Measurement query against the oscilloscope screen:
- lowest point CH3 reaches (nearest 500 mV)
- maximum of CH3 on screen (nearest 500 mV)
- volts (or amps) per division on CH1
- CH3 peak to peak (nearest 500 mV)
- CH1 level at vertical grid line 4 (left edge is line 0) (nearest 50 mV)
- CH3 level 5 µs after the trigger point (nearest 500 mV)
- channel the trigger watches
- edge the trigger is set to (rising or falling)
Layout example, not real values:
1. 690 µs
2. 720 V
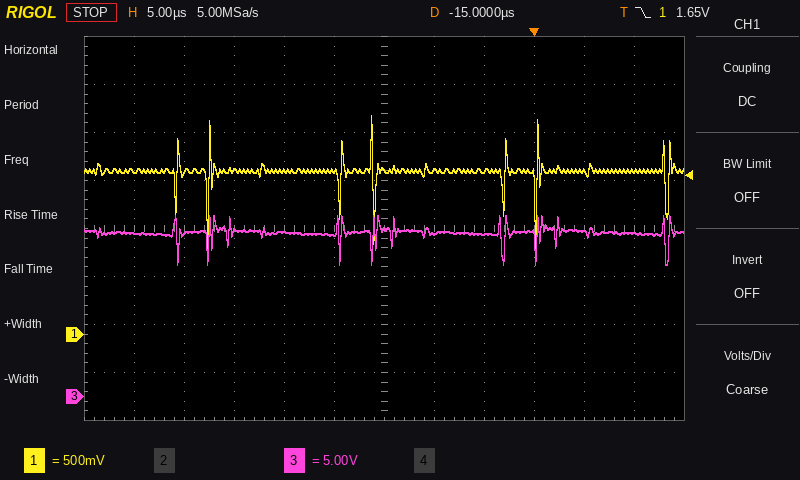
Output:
1. 14.0 V
2. 19.0 V
3. 500 mV
4. 5.0 V
5. 1.70 V
6. 17.0 V
7. CH1
8. falling
